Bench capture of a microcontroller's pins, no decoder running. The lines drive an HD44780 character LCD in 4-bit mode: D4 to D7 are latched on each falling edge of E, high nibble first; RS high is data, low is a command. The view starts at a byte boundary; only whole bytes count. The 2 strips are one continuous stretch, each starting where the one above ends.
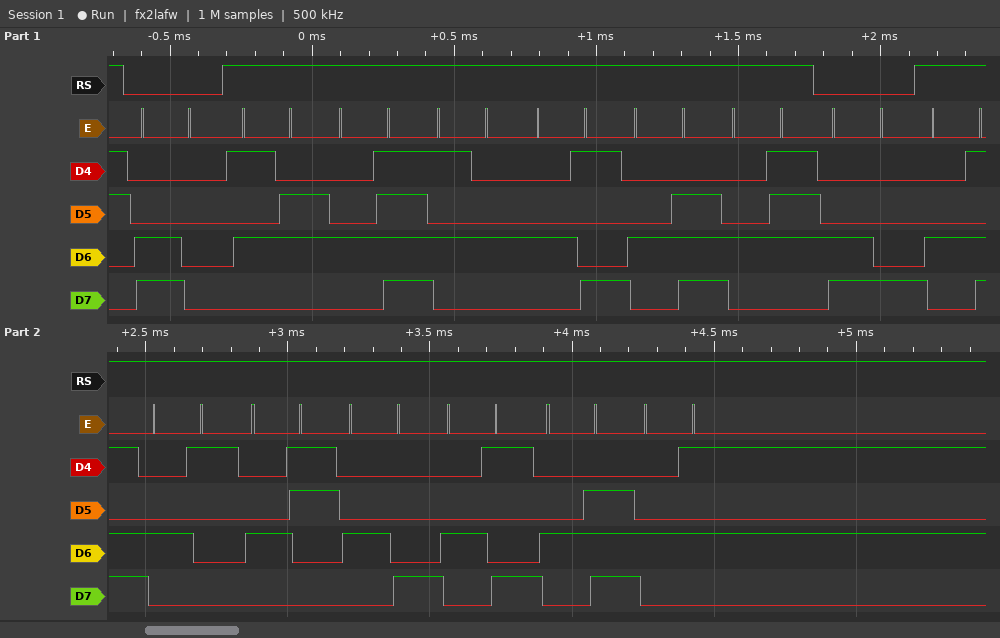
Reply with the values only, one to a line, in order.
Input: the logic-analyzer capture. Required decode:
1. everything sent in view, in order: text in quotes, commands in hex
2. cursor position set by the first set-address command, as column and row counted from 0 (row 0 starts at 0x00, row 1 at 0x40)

0xC0 "VOTING" 0xC8 "MACHINE"
column 0, row 1
